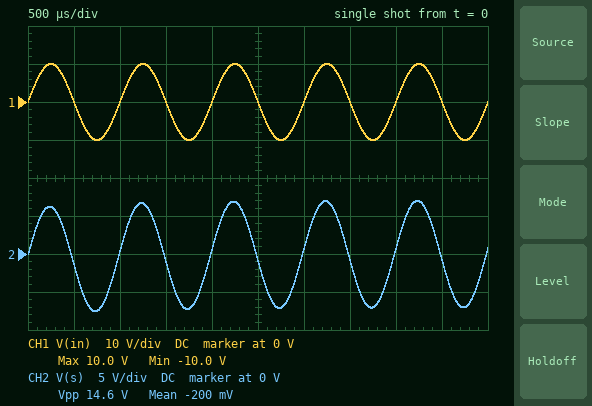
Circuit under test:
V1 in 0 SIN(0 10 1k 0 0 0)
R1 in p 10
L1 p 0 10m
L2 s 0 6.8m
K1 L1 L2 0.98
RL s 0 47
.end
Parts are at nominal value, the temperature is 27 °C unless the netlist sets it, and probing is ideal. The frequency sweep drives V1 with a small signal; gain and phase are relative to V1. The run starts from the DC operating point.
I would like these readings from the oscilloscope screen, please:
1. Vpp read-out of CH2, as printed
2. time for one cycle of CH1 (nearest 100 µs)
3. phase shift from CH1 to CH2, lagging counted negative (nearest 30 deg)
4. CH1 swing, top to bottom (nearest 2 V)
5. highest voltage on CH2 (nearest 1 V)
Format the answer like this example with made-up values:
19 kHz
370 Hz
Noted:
14.6 V
1.0 ms
0 deg
20 V
7 V
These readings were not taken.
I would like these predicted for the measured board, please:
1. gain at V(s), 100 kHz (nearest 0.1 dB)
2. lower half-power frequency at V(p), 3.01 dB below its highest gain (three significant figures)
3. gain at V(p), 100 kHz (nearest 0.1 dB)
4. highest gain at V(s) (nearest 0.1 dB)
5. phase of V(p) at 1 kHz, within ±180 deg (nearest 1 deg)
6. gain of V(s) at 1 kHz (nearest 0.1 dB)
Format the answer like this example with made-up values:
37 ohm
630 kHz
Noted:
-13.4 dB
190 Hz
-0.1 dB
-3.0 dB
8 deg
-3.1 dB
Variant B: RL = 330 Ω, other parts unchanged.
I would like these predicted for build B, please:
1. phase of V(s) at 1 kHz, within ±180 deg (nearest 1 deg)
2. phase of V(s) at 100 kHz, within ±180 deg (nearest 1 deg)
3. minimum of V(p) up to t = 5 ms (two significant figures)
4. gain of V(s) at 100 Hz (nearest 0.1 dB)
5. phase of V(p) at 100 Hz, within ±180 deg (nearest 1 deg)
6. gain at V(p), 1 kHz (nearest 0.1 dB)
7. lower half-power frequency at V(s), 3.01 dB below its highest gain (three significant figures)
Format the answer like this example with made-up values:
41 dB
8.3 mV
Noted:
9 deg
-27 deg
-10 V
-7.4 dB
57 deg
-0.3 dB
156 Hz
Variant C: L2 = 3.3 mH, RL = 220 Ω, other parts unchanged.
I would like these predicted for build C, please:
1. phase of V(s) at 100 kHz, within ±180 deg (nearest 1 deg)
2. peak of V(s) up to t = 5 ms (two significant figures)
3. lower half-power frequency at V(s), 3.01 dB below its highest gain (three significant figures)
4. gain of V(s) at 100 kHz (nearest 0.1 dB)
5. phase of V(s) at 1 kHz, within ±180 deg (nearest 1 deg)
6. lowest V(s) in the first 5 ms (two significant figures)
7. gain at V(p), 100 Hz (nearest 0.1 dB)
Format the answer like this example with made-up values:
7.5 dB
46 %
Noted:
-20 deg
5.5 V
157 Hz
-5.7 dB
9 deg
-5.9 V
-5.5 dB
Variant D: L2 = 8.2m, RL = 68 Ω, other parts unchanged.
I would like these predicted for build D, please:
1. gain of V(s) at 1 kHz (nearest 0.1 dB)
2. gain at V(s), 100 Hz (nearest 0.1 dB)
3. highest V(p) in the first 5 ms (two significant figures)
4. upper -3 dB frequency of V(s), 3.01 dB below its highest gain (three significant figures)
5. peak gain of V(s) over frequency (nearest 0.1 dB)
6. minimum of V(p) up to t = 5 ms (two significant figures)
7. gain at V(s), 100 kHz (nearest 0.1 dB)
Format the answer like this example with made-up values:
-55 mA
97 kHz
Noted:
-2.1 dB
-6.8 dB
8.8 V
37.5 kHz
-2.0 dB
-9.5 V
-11.1 dB
